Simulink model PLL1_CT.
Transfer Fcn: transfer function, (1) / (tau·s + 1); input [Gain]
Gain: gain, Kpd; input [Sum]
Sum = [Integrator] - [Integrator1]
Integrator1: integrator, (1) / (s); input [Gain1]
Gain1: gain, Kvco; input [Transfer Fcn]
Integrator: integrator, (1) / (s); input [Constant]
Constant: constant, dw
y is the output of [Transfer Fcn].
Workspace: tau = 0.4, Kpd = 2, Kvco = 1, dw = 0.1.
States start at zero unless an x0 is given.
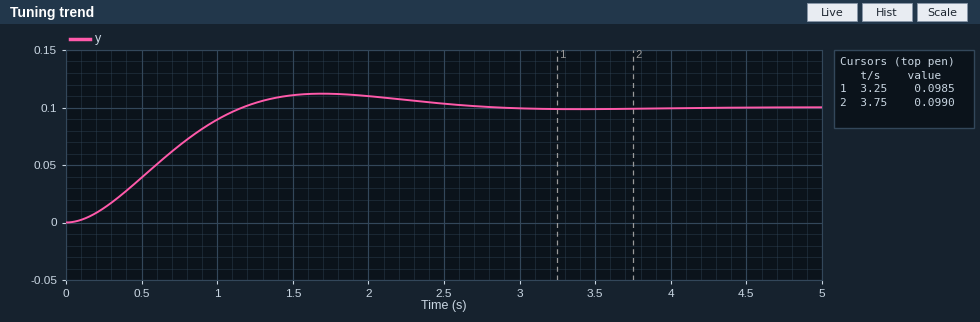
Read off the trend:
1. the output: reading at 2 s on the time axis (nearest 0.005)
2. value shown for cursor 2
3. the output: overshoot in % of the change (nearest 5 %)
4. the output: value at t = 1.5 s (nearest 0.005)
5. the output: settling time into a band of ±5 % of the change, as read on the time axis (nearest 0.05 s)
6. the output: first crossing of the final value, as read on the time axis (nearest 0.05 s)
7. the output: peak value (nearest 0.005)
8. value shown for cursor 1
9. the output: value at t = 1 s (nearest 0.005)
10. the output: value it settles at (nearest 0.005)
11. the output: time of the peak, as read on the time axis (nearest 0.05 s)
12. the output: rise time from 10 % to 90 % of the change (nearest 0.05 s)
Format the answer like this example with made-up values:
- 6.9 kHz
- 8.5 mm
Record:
- 0.110
- 0.0990
- 10 %
- 0.110
- 2.35 s
- 1.15 s
- 0.110
- 0.0985
- 0.090
- 0.100
- 1.70 s
- 0.80 s
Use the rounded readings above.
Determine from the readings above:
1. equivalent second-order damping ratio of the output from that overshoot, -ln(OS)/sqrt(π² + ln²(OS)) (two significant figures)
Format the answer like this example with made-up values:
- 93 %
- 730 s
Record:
- 0.59
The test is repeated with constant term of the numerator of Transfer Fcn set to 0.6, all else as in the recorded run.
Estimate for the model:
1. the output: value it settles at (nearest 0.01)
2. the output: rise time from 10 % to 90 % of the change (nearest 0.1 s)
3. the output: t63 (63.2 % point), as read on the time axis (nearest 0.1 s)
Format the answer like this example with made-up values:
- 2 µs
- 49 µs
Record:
- 0.10
- 1.3 s
- 1.0 s
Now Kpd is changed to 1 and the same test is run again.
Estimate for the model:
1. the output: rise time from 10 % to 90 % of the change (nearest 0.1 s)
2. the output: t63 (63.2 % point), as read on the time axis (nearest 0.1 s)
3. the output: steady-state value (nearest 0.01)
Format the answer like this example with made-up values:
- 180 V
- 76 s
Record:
- 1.5 s
- 1.2 s
- 0.10
